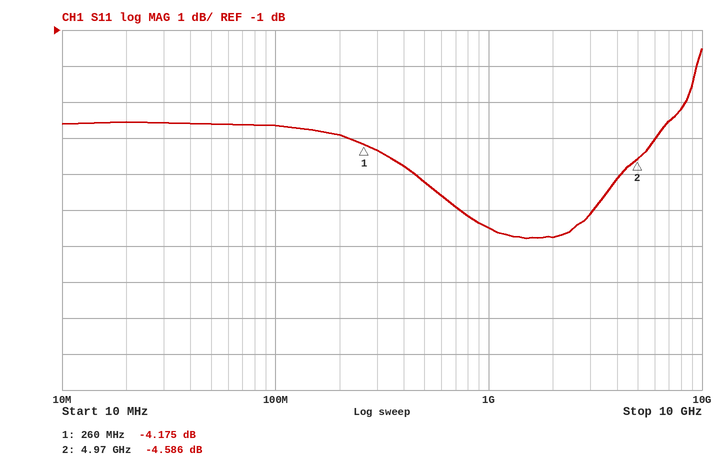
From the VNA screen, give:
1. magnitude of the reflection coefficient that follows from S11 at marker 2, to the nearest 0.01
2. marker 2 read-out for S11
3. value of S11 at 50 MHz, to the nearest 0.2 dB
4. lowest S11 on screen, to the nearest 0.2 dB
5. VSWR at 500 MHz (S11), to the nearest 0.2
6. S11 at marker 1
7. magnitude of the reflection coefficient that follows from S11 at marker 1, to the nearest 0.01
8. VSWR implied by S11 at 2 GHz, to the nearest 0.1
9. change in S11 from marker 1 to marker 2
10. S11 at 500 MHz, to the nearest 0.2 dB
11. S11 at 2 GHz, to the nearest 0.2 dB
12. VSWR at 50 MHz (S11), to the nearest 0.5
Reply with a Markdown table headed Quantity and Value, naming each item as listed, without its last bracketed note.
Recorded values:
| Quantity | Value |
|---|---|
| magnitude of the reflection coefficient that follows from S11 at marker 2, to the nearest 0.01 | 0.59 |
| marker 2 read-out for S11 | -4.586 dB |
| value of S11 at 50 MHz, to the nearest 0.2 dB | -3.6 dB |
| lowest S11 on screen, to the nearest 0.2 dB | -6.8 dB |
| VSWR at 500 MHz (S11), to the nearest 0.2 | 3.4 |
| S11 at marker 1 | -4.175 dB |
| magnitude of the reflection coefficient that follows from S11 at marker 1, to the nearest 0.01 | 0.62 |
| VSWR implied by S11 at 2 GHz, to the nearest 0.1 | 2.7 |
| change in S11 from marker 1 to marker 2 | -0.411 dB |
| S11 at 500 MHz, to the nearest 0.2 dB | -5.2 dB |
| S11 at 2 GHz, to the nearest 0.2 dB | -6.8 dB |
| VSWR at 50 MHz (S11), to the nearest 0.5 | 5.0 |
